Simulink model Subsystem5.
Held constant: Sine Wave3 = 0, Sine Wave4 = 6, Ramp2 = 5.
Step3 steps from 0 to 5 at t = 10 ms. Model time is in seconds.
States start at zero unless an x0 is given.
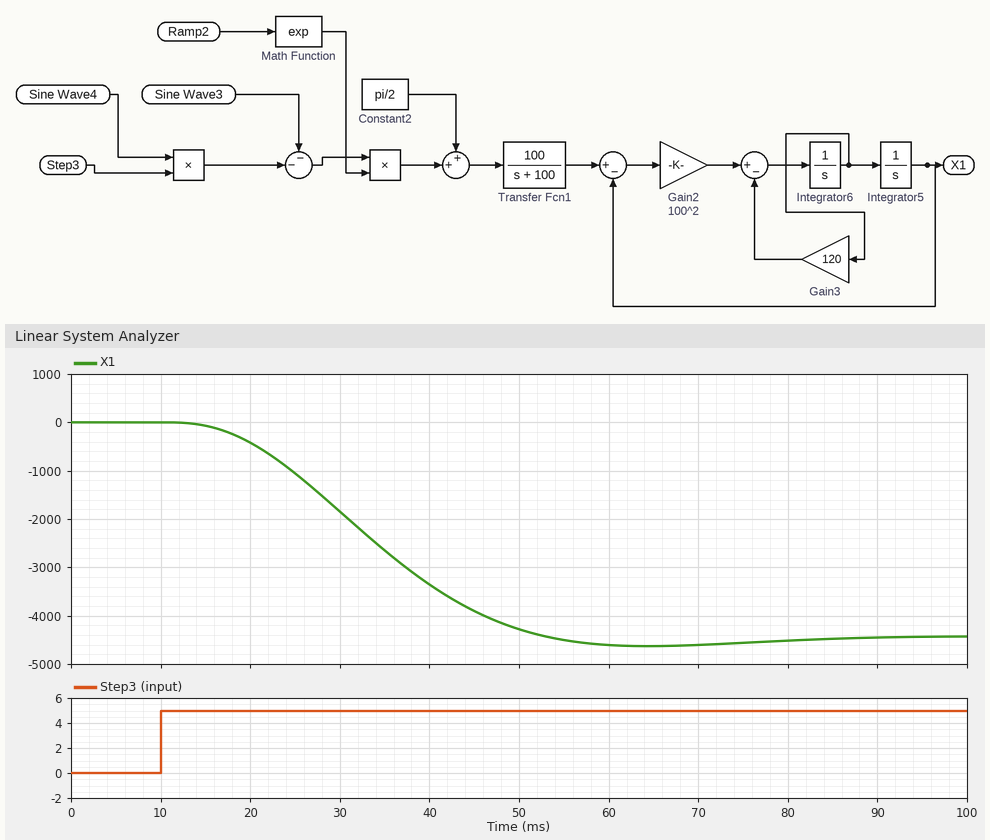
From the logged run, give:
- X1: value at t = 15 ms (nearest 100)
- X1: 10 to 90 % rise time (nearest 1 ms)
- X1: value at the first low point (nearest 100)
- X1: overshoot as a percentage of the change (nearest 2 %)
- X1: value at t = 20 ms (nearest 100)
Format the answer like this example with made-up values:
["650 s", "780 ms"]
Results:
["-100", "26 ms", "-4600", "4 %", "-400"]
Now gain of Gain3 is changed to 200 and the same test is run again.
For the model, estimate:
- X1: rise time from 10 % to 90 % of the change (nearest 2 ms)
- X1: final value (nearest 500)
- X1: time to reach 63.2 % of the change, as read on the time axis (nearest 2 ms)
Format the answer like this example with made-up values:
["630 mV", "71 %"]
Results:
["42 ms", "-4500", "42 ms"]
